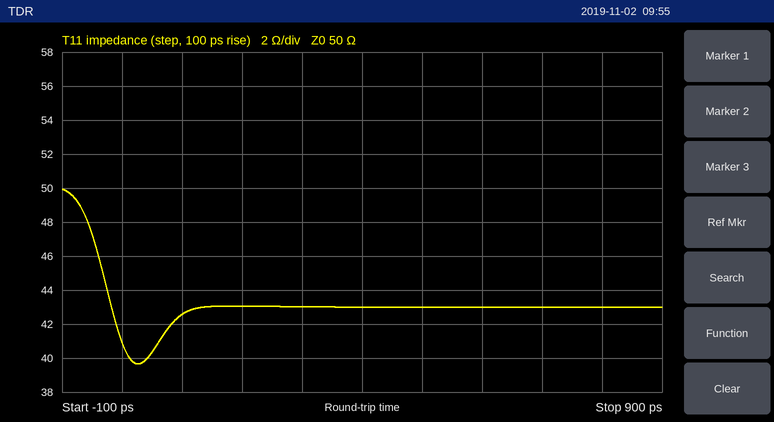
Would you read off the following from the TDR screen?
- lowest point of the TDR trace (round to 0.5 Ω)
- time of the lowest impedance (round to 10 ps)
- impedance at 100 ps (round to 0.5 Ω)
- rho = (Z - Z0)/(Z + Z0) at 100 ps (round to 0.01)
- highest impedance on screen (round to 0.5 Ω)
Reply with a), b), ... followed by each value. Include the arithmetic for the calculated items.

a) 39.5 Ω
b) 30 ps
c) 42.5 Ω
d) (42.5 − 50)/(42.5 + 50) ≈ -0.08
e) 50.0 Ω
